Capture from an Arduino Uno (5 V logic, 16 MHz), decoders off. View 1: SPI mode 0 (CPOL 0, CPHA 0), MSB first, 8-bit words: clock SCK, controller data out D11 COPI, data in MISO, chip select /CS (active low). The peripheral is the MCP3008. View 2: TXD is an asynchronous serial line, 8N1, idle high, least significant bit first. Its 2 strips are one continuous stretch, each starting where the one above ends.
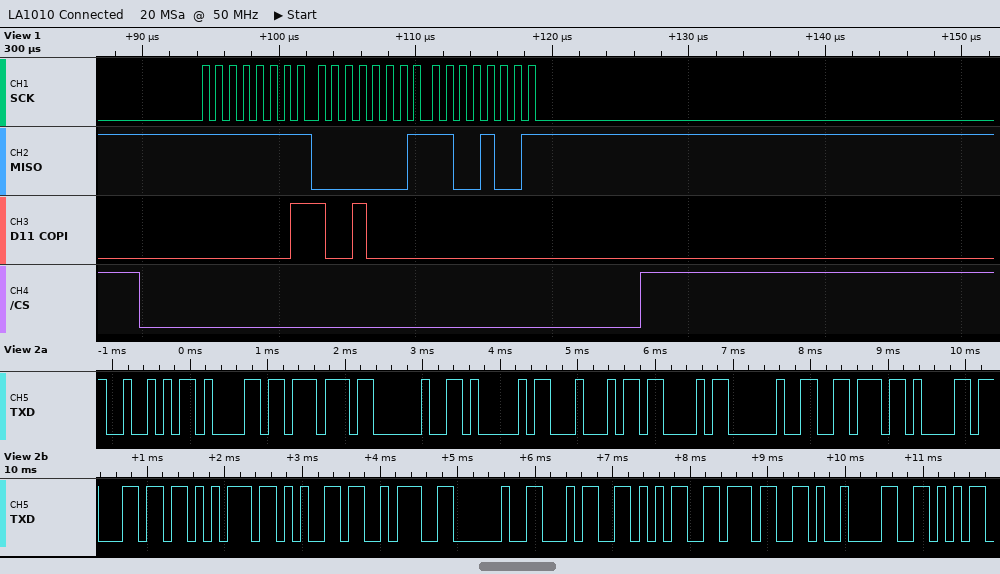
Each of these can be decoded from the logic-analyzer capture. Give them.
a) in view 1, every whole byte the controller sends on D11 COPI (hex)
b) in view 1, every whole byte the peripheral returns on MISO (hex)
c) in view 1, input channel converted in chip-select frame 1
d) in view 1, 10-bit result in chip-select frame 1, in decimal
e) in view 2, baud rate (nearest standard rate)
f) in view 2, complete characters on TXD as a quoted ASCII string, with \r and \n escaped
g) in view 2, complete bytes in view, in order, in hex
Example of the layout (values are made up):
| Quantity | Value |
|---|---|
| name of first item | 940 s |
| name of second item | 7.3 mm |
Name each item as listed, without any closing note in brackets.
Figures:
| Quantity | Value |
|---|---|
| in view 1, every whole byte the controller sends on D11 COPI | 0x01 0x90 0x00 |
| in view 1, every whole byte the peripheral returns on MISO | 0xFF 0x01 0xC9 |
| in view 1, input channel converted in chip-select frame 1 | 1 |
| in view 1, 10-bit result in chip-select frame 1, in decimal | 457 |
| in view 2, baud rate | 9600 baud |
| in view 2, complete characters on TXD as a quoted ASCII string, with \r and \n escaped | "Raw ADC value: 457\tV" |
| in view 2, complete bytes in view, in order, in hex | 0x52 0x61 0x77 0x20 0x41 0x44 0x43 0x20 0x76 0x61 0x6C 0x75 0x65 0x3A 0x20 0x34 0x35 0x37 0x09 0x56 |
